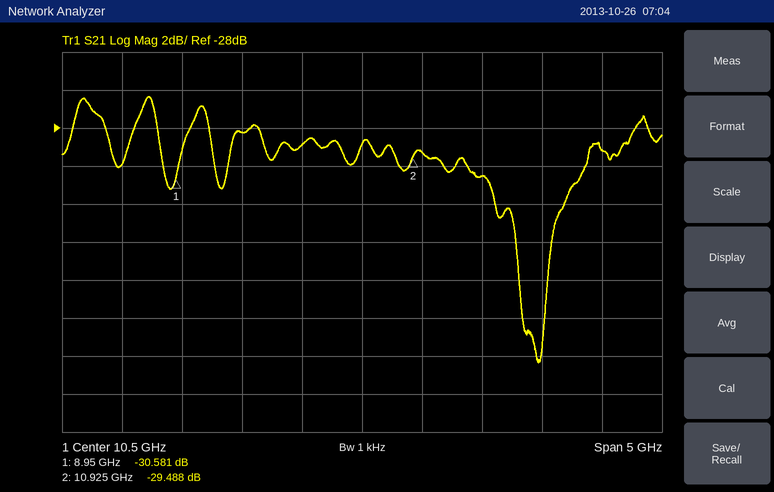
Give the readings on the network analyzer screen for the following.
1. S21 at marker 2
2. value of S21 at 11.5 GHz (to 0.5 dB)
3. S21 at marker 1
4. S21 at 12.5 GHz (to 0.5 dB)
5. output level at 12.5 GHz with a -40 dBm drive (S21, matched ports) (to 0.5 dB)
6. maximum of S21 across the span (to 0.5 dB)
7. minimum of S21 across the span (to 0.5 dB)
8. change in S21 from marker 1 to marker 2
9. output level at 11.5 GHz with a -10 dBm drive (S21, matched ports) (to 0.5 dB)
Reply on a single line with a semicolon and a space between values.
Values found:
-29.488 dB; -30.5 dB; -30.581 dB; -29.0 dB; -69.0 dBm; -26.5 dB; -40.5 dB; 1.093 dB; -40.5 dBm
